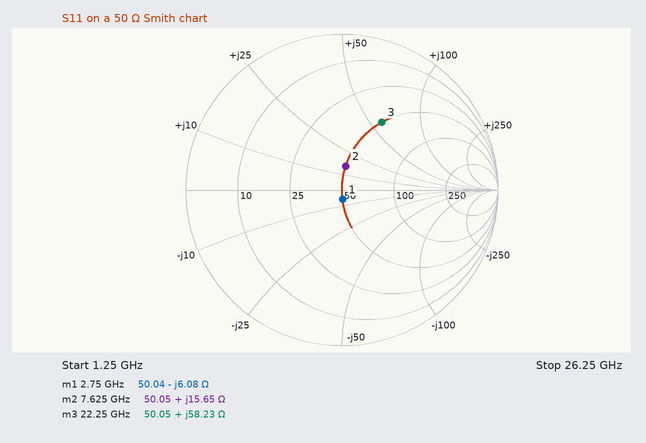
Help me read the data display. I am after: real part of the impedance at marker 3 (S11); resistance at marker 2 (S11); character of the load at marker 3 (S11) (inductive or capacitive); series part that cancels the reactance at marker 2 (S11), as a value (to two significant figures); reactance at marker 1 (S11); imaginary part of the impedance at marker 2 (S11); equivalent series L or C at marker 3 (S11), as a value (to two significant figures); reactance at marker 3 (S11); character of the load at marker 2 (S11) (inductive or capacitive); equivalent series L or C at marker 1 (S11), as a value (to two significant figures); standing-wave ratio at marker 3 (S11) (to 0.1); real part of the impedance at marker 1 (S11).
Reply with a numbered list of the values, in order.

1. 50.05 Ω
2. 50.05 Ω
3. inductive
4. 1.3 pF
5. -6.08 Ω
6. +15.65 Ω
7. 420 pH
8. +58.23 Ω
9. inductive
10. 9.5 pF
11. 3.0
12. 50.04 Ω
